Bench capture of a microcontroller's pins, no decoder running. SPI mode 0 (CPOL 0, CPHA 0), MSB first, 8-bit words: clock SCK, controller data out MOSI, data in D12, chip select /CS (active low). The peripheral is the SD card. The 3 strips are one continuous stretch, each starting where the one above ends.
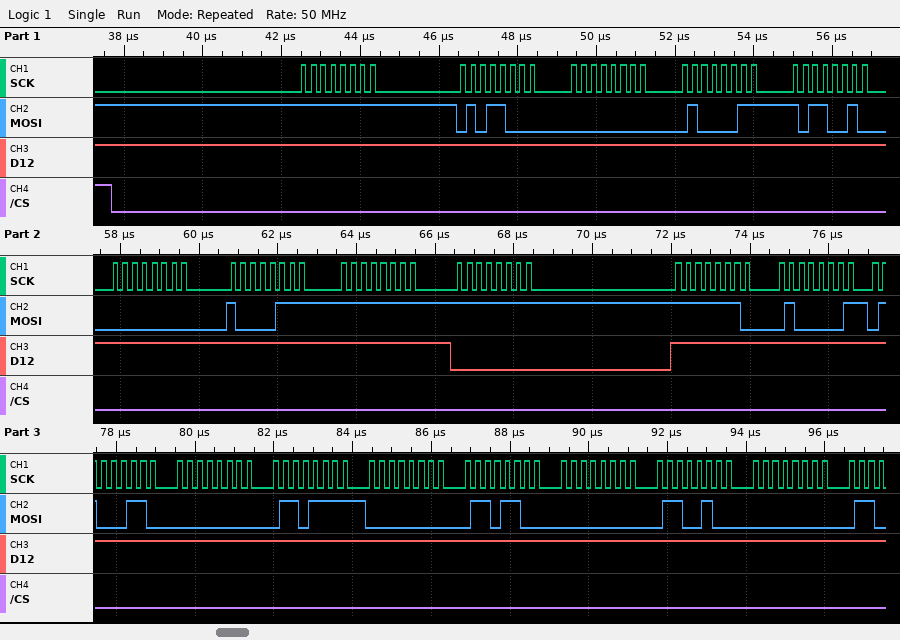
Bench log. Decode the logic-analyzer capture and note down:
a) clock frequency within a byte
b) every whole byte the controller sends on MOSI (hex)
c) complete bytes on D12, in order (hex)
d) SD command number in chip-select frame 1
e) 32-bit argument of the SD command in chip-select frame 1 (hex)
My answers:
4 MHz
FF 58 00 43 B2 00 87 FF FF FE 41 46 00 6F 00 6C 00 64 00
FF FF FF FF FF FF FF FF 00 FF FF FF FF FF FF FF FF FF FF
CMD24
0x0043B200
